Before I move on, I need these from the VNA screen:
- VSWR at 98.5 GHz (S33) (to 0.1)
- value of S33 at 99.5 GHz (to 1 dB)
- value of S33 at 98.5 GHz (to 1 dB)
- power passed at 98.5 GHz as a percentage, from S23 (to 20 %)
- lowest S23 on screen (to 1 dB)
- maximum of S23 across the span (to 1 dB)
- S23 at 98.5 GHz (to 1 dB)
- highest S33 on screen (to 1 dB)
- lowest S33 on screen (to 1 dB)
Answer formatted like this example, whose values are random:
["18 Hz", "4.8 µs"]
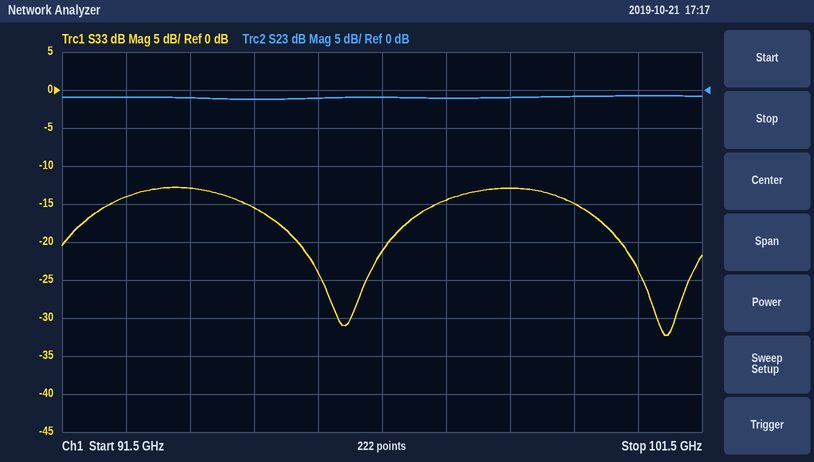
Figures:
["1.6", "-15 dB", "-13 dB", "80 %", "-1 dB", "-1 dB", "-1 dB", "-13 dB", "-32 dB"]
